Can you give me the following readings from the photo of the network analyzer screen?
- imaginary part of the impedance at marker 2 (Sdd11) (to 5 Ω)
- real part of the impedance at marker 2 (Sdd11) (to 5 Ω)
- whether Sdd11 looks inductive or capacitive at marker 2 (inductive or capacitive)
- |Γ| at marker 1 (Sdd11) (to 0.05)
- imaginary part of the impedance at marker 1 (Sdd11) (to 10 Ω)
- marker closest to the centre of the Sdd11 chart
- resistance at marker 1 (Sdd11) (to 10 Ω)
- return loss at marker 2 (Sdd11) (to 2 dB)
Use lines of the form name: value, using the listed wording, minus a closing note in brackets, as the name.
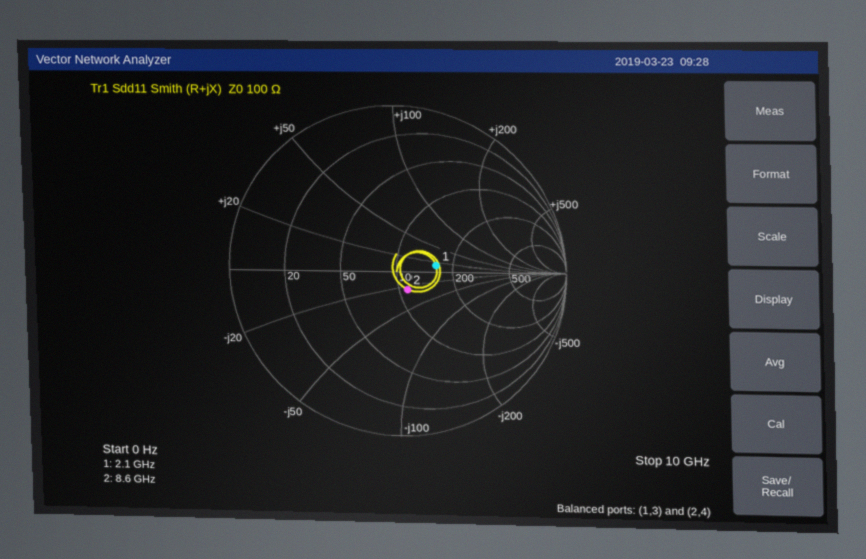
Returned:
imaginary part of the impedance at marker 2 (Sdd11): -25 Ω
real part of the impedance at marker 2 (Sdd11): 110 Ω
whether Sdd11 looks inductive or capacitive at marker 2: capacitive
|Γ| at marker 1 (Sdd11): 0.25
imaginary part of the impedance at marker 1 (Sdd11): +10 Ω
marker closest to the centre of the Sdd11 chart: marker 2
resistance at marker 1 (Sdd11): 160 Ω
return loss at marker 2 (Sdd11): 18 dB
